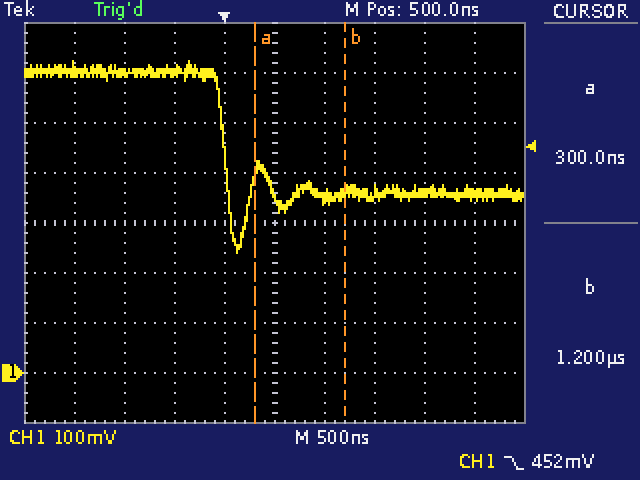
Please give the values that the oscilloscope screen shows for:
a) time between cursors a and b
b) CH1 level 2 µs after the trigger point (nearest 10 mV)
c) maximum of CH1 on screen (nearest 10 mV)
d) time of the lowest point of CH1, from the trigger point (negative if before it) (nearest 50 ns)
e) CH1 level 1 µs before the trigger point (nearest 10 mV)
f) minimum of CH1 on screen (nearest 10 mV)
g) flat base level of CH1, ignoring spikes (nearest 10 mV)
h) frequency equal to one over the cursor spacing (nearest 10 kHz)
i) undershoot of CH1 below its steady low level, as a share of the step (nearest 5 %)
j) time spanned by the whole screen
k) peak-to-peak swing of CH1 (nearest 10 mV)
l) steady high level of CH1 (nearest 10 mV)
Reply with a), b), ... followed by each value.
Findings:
a) 900 ns
b) 360 mV
c) 620 mV
d) +150 ns
e) 600 mV
f) 240 mV
g) 360 mV
h) 1.11 MHz
i) 50 %
j) 5 µs
k) 380 mV
l) 600 mV
